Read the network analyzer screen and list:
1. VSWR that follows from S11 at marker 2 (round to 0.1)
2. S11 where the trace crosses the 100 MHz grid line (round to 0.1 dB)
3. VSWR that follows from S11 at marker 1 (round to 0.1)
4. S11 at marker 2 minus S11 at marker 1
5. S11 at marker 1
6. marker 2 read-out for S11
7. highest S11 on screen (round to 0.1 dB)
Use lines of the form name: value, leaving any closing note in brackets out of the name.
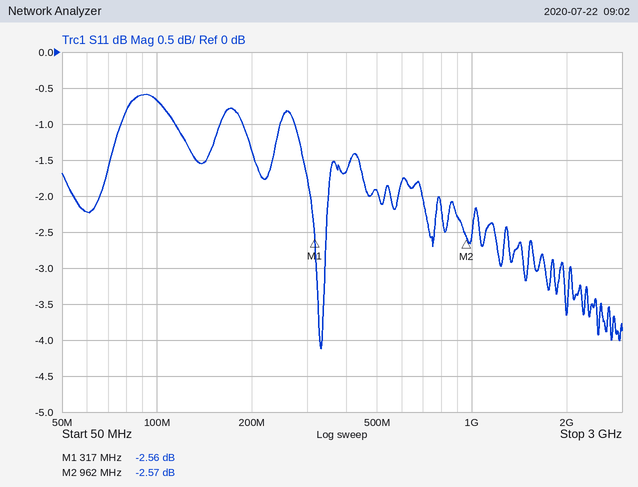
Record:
VSWR that follows from S11 at marker 2: 6.8
S11 where the trace crosses the 100 MHz grid line: -0.7 dB
VSWR that follows from S11 at marker 1: 6.8
S11 at marker 2 minus S11 at marker 1: -0.01 dB
S11 at marker 1: -2.56 dB
marker 2 read-out for S11: -2.57 dB
highest S11 on screen: -0.6 dB
